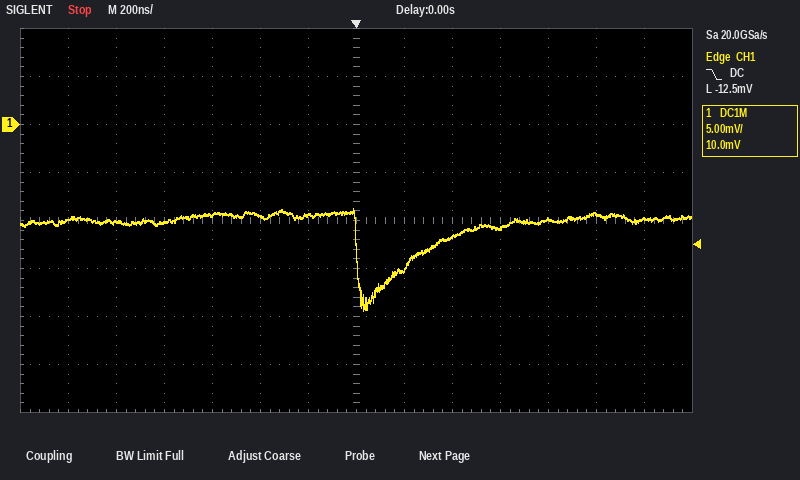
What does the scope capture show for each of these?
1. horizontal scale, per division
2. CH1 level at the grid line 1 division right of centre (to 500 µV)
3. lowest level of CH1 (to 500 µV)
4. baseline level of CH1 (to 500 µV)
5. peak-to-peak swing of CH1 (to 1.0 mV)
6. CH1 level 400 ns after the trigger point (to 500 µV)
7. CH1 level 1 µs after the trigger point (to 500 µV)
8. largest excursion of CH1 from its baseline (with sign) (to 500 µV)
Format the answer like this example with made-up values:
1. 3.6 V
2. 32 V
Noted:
1. 200 ns
2. -15.0 mV
3. -19.5 mV
4. -10.0 mV
5. 11.0 mV
6. -11.5 mV
7. -9.5 mV
8. -9.5 mV
